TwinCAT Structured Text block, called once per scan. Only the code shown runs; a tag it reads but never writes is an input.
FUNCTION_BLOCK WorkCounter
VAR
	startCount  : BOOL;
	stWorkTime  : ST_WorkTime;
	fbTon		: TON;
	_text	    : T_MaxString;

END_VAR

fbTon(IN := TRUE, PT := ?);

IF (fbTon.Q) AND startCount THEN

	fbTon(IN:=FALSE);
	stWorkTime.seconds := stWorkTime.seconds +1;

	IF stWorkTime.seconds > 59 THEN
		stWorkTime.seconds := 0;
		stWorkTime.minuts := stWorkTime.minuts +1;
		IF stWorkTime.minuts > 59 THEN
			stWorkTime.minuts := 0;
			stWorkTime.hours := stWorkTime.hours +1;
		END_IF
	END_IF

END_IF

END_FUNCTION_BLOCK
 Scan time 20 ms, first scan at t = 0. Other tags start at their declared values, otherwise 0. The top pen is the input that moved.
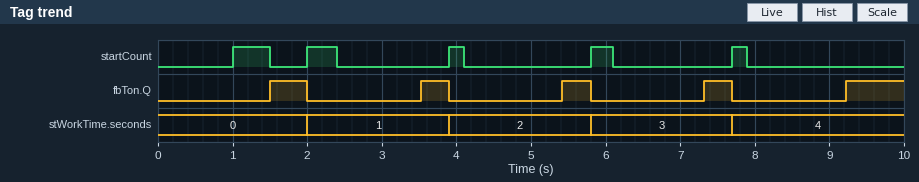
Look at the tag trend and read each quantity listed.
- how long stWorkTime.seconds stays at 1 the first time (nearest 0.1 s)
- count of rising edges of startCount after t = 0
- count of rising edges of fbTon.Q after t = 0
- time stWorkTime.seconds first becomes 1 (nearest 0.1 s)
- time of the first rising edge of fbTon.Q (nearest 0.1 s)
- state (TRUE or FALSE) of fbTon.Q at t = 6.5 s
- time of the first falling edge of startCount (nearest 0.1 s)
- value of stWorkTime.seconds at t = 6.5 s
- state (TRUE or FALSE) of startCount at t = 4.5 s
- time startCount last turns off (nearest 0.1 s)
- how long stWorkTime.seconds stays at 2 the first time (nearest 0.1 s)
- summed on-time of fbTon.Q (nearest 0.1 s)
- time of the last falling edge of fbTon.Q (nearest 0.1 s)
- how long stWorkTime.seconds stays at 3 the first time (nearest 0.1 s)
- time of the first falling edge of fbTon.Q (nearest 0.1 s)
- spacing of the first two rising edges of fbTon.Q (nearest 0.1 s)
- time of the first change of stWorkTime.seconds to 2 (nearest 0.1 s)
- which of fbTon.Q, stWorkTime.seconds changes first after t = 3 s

1.9 s
5
5
2.0 s
1.5 s
FALSE
1.5 s
3
FALSE
7.9 s
1.9 s
2.4 s
7.7 s
1.9 s
2.0 s
2.0 s
3.9 s
fbTon.Q
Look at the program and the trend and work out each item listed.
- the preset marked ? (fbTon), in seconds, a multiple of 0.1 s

1.5 s
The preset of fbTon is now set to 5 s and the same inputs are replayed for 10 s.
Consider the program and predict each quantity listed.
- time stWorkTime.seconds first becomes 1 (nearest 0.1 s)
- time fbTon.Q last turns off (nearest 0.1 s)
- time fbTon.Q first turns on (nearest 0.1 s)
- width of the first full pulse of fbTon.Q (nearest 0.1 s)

5.8 s
5.8 s
5.0 s
0.8 s
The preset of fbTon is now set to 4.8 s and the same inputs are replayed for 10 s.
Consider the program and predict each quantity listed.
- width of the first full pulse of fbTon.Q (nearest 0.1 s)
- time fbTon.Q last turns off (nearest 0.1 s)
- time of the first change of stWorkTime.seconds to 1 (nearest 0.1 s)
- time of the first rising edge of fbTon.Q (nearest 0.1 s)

1.0 s
5.8 s
5.8 s
4.8 s
